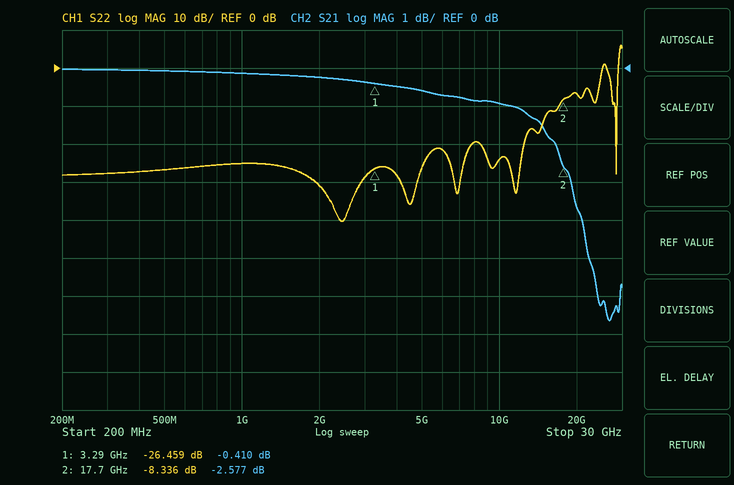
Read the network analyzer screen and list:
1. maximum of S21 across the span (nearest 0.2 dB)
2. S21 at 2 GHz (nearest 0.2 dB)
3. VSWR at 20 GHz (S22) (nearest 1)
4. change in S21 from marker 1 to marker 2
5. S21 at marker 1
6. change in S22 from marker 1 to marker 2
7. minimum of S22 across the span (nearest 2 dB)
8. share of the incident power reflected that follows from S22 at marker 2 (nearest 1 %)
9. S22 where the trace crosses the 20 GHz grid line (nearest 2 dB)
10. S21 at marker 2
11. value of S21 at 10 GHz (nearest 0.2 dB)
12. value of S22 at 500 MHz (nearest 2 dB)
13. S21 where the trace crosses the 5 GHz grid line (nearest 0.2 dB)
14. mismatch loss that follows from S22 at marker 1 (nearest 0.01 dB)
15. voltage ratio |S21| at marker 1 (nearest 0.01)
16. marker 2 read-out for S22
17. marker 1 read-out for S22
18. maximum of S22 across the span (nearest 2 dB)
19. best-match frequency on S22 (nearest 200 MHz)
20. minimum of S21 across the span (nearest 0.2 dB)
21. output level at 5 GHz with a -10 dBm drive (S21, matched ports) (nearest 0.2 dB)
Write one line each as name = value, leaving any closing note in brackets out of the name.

maximum of S21 across the span = 0.0 dB
S21 at 2 GHz = -0.2 dB
VSWR at 20 GHz (S22) = 3
change in S21 from marker 1 to marker 2 = -2.167 dB
S21 at marker 1 = -0.410 dB
change in S22 from marker 1 to marker 2 = 18.123 dB
minimum of S22 across the span = -40 dB
share of the incident power reflected that follows from S22 at marker 2 = 15 %
S22 where the trace crosses the 20 GHz grid line = -6 dB
S21 at marker 2 = -2.577 dB
value of S21 at 10 GHz = -1.0 dB
value of S22 at 500 MHz = -26 dB
S21 where the trace crosses the 5 GHz grid line = -0.6 dB
mismatch loss that follows from S22 at marker 1 = 0.01 dB
voltage ratio |S21| at marker 1 = 0.95
marker 2 read-out for S22 = -8.336 dB
marker 1 read-out for S22 = -26.459 dB
maximum of S22 across the span = 6 dB
best-match frequency on S22 = 2.4 GHz
minimum of S21 across the span = -6.6 dB
output level at 5 GHz with a -10 dBm drive (S21, matched ports) = -10.6 dBm
